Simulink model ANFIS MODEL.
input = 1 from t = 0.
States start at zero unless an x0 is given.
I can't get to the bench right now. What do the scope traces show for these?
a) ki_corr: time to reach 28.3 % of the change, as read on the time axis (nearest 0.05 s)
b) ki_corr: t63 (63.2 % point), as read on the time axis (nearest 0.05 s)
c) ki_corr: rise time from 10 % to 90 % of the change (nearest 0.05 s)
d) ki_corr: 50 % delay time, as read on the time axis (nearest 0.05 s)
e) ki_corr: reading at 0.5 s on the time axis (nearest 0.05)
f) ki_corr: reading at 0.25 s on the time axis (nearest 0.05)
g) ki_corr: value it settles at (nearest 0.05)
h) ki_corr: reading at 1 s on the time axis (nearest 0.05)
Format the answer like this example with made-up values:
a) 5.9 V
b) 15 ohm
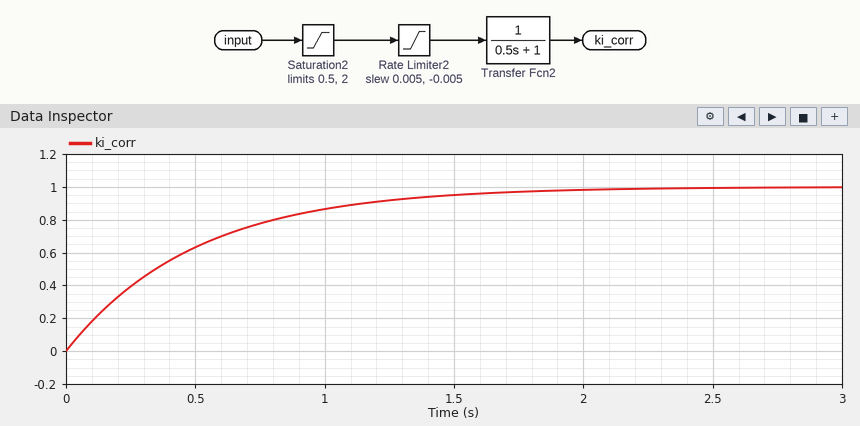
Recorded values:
a) 0.15 s
b) 0.50 s
c) 1.10 s
d) 0.35 s
e) 0.65
f) 0.40
g) 1.00
h) 0.85
